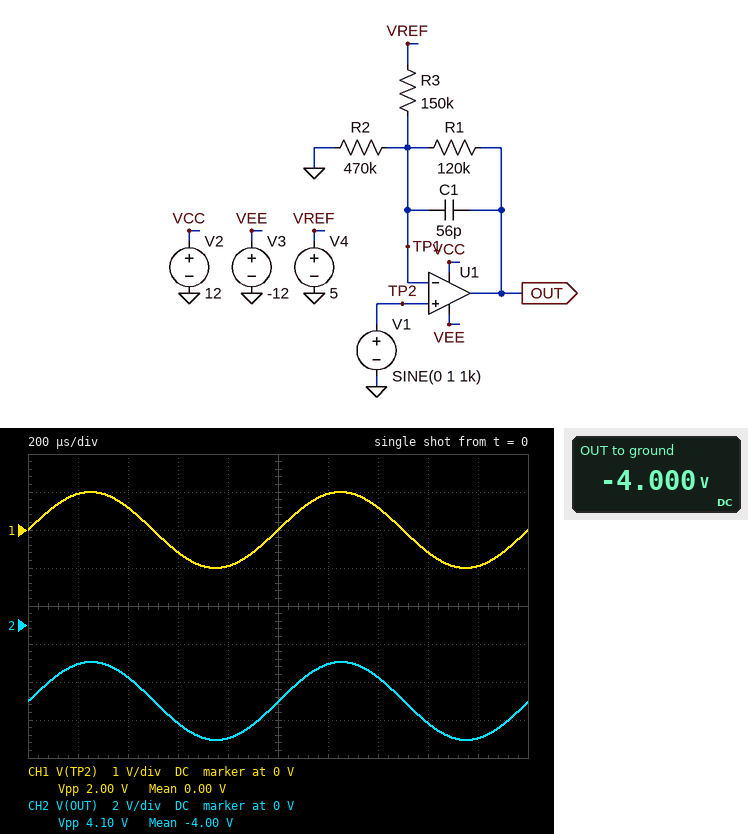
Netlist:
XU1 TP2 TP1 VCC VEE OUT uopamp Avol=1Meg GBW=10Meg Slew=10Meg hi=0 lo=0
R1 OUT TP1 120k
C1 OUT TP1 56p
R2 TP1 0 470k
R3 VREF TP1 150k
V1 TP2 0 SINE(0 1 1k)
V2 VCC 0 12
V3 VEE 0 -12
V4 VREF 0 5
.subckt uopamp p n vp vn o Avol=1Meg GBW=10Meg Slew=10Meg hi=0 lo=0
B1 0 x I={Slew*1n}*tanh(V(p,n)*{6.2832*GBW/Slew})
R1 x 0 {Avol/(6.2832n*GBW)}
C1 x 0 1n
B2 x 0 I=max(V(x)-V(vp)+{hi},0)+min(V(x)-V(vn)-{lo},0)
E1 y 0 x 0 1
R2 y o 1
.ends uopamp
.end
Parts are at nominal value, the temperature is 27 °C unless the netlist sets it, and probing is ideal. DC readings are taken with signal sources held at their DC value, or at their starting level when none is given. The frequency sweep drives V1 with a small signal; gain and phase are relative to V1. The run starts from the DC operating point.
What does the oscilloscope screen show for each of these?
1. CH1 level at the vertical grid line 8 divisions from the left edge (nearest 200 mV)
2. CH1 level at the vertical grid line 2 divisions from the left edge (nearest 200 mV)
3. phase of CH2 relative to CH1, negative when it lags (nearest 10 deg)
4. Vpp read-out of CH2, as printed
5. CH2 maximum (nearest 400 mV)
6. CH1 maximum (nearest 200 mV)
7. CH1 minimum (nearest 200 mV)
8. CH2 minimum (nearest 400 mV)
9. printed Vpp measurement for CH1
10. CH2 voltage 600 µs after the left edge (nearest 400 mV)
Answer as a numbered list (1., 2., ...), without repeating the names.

1. -600 mV
2. 600 mV
3. 0 deg
4. 4.10 V
5. -2.0 V
6. 1.0 V
7. -1.0 V
8. -6.0 V
9. 2.00 V
10. -5.2 V
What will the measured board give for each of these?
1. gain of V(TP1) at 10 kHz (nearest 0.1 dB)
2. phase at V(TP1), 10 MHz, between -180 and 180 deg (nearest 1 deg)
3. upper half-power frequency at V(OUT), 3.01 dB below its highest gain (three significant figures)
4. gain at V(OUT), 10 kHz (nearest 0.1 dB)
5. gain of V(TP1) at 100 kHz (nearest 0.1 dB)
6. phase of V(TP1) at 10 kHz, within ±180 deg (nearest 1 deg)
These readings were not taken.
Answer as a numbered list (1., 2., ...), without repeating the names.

1. 0 dB
2. -45 deg
3. 32.5 kHz
4. 5.7 dB
5. 0 dB
6. 0 deg
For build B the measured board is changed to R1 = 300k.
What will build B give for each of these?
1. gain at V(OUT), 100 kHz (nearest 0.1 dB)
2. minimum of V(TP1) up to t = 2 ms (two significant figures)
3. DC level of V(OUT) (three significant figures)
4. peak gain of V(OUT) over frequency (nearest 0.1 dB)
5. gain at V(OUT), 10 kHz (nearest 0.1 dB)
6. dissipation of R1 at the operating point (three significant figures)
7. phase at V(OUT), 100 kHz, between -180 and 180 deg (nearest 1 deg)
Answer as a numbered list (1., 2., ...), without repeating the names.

1. 0.4 dB
2. -610 mV
3. -10.0 V
4. 11.2 dB
5. 8.3 dB
6. 333 µW
7. -14 deg
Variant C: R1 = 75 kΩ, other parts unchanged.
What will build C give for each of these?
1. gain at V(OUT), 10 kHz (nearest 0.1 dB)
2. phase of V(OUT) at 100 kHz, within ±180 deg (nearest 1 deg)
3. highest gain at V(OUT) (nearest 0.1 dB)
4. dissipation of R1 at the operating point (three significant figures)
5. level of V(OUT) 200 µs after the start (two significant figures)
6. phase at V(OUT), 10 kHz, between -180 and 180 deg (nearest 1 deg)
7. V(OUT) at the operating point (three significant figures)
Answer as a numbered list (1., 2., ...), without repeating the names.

1. 4.2 dB
2. -12 deg
3. 4.4 dB
4. 83.3 µW
5. -930 mV
6. -6 deg
7. -2.50 V
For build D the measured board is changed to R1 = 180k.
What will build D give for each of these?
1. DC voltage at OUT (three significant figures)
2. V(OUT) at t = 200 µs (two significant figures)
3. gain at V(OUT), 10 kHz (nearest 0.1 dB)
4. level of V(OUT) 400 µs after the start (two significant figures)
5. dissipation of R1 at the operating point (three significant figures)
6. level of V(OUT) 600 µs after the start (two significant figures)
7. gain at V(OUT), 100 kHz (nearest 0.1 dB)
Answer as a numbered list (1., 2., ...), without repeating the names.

1. -6.00 V
2. -3.6 V
3. 7.0 dB
4. -4.4 V
5. 200 µW
6. -7.4 V
7. 0.5 dB
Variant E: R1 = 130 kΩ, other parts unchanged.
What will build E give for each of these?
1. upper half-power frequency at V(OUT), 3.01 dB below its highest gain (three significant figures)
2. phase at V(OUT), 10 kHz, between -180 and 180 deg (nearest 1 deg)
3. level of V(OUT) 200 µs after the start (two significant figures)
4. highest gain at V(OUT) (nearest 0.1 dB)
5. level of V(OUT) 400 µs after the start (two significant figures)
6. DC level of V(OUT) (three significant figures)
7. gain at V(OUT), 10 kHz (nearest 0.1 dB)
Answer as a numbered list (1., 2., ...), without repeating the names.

1. 29.0 kHz
2. -13 deg
3. -2.3 V
4. 6.6 dB
5. -3.0 V
6. -4.33 V
7. 6.0 dB
